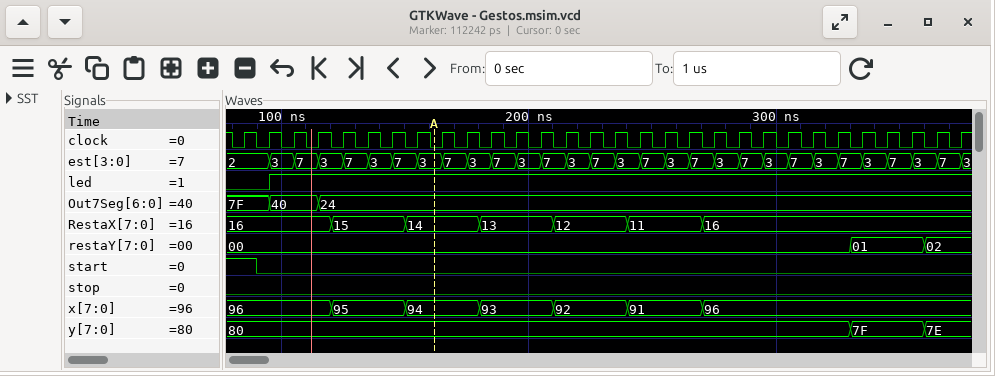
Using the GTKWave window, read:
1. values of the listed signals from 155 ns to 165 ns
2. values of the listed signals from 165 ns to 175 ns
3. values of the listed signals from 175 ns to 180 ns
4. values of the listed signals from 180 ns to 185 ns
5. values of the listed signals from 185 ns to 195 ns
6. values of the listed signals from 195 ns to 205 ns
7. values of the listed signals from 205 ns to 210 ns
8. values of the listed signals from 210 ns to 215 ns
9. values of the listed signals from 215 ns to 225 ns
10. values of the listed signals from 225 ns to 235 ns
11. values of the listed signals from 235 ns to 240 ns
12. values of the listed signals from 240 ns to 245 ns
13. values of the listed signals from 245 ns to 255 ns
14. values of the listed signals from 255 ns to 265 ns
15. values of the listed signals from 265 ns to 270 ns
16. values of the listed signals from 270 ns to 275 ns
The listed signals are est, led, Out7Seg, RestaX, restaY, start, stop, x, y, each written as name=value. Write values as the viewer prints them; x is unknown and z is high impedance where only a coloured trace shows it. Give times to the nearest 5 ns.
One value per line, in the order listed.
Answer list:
est=3, led=1, Out7Seg=24, RestaX=14, restaY=00, start=0, stop=0, x=94, y=80
est=7, led=1, Out7Seg=24, RestaX=14, restaY=00, start=0, stop=0, x=94, y=80
est=3, led=1, Out7Seg=24, RestaX=14, restaY=00, start=0, stop=0, x=94, y=80
est=3, led=1, Out7Seg=24, RestaX=13, restaY=00, start=0, stop=0, x=93, y=80
est=7, led=1, Out7Seg=24, RestaX=13, restaY=00, start=0, stop=0, x=93, y=80
est=3, led=1, Out7Seg=24, RestaX=13, restaY=00, start=0, stop=0, x=93, y=80
est=7, led=1, Out7Seg=24, RestaX=13, restaY=00, start=0, stop=0, x=93, y=80
est=7, led=1, Out7Seg=24, RestaX=12, restaY=00, start=0, stop=0, x=92, y=80
est=3, led=1, Out7Seg=24, RestaX=12, restaY=00, start=0, stop=0, x=92, y=80
est=7, led=1, Out7Seg=24, RestaX=12, restaY=00, start=0, stop=0, x=92, y=80
est=3, led=1, Out7Seg=24, RestaX=12, restaY=00, start=0, stop=0, x=92, y=80
est=3, led=1, Out7Seg=24, RestaX=11, restaY=00, start=0, stop=0, x=91, y=80
est=7, led=1, Out7Seg=24, RestaX=11, restaY=00, start=0, stop=0, x=91, y=80
est=3, led=1, Out7Seg=24, RestaX=11, restaY=00, start=0, stop=0, x=91, y=80
est=7, led=1, Out7Seg=24, RestaX=11, restaY=00, start=0, stop=0, x=91, y=80
est=7, led=1, Out7Seg=24, RestaX=16, restaY=00, start=0, stop=0, x=96, y=80
